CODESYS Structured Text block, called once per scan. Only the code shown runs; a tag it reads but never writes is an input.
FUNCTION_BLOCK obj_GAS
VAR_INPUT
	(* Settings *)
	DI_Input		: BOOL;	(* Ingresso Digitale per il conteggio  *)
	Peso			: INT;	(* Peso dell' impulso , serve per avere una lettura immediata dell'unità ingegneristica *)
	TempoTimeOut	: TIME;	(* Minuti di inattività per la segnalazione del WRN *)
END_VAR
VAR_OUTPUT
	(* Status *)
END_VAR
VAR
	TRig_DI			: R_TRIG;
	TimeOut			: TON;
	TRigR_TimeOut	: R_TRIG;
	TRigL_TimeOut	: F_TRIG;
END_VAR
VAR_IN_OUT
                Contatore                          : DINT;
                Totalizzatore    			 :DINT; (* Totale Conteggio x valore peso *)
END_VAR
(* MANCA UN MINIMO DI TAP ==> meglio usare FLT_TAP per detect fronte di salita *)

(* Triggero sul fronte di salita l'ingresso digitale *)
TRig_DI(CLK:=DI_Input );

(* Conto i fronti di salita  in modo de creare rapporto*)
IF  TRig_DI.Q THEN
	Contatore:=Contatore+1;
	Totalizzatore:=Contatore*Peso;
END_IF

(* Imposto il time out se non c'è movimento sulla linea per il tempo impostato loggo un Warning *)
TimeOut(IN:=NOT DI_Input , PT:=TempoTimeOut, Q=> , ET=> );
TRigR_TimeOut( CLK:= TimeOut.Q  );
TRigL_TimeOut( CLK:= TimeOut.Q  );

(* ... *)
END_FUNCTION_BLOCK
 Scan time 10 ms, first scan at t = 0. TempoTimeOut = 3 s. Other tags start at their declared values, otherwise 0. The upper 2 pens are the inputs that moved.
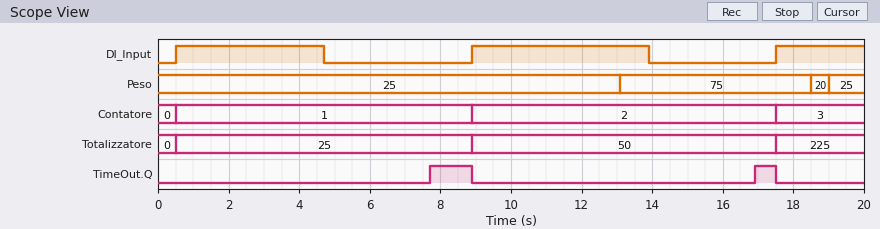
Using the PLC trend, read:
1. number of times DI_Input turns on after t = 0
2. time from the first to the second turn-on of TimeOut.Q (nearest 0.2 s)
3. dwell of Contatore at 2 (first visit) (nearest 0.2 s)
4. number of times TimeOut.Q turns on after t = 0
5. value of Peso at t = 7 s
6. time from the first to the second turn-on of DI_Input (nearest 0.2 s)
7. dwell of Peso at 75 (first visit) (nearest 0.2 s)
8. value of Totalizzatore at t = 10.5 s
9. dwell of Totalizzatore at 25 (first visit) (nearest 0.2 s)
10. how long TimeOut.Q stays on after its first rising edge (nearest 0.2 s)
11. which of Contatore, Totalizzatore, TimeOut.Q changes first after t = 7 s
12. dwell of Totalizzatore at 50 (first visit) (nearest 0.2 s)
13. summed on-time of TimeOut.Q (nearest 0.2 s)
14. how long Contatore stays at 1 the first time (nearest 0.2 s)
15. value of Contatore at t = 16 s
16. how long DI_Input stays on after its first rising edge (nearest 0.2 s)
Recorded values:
3
9.2 s
8.6 s
2
25
8.4 s
5.4 s
50
8.4 s
1.2 s
TimeOut.Q
8.6 s
1.8 s
8.4 s
2
4.2 s
